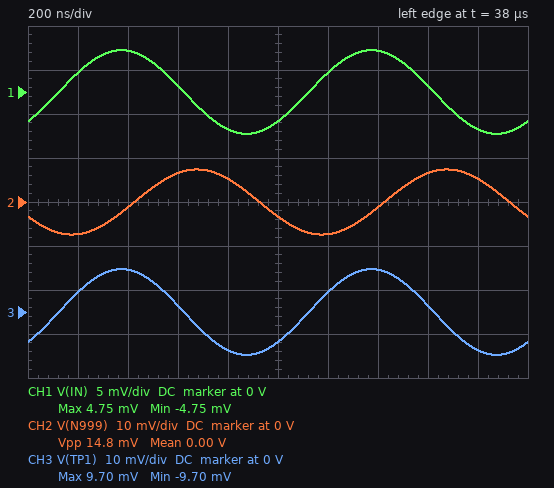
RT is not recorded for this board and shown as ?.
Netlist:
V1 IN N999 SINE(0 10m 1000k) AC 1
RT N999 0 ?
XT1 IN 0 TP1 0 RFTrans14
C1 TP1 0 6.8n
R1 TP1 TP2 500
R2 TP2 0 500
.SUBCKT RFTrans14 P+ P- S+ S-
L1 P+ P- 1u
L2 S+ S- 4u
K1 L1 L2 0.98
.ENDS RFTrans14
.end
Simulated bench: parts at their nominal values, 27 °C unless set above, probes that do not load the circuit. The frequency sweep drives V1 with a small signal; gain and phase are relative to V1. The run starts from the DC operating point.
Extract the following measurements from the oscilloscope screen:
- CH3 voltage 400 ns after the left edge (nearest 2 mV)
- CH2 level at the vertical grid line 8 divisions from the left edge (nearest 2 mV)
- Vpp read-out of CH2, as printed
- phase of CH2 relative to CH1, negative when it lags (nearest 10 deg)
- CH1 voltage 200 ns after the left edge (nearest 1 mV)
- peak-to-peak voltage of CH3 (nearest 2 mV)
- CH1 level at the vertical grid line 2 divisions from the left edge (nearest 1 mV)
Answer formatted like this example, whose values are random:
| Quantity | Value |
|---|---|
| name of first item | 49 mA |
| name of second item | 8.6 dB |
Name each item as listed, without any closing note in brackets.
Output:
| Quantity | Value |
|---|---|
| CH3 voltage 400 ns after the left edge | 10 mV |
| CH2 level at the vertical grid line 8 divisions from the left edge | 6 mV |
| Vpp read-out of CH2, as printed | 14.8 mV |
| phase of CH2 relative to CH1, negative when it lags | -110 deg |
| CH1 voltage 200 ns after the left edge | 2 mV |
| peak-to-peak voltage of CH3 | 20 mV |
| CH1 level at the vertical grid line 2 divisions from the left edge | 5 mV |
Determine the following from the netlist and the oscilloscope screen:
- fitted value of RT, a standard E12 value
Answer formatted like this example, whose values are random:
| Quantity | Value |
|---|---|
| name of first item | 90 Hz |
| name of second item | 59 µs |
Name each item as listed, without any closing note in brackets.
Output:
| Quantity | Value |
|---|---|
| fitted value of RT, a standard E12 value | 120 Ω |
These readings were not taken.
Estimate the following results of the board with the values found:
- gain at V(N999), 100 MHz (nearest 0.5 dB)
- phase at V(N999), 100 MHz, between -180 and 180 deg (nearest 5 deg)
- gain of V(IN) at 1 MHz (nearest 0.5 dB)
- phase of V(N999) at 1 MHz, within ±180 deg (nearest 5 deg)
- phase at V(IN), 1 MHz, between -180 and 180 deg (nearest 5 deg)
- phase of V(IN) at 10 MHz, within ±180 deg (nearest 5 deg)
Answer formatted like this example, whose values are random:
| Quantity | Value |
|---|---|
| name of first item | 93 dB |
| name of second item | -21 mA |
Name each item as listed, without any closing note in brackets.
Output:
| Quantity | Value |
|---|---|
| gain at V(N999), 100 MHz | 0 dB |
| phase at V(N999), 100 MHz, between -180 and 180 deg | 170 deg |
| gain of V(IN) at 1 MHz | -6.5 dB |
| phase of V(N999) at 1 MHz, within ±180 deg | -155 deg |
| phase at V(IN), 1 MHz, between -180 and 180 deg | -45 deg |
| phase of V(IN) at 10 MHz, within ±180 deg | 90 deg |
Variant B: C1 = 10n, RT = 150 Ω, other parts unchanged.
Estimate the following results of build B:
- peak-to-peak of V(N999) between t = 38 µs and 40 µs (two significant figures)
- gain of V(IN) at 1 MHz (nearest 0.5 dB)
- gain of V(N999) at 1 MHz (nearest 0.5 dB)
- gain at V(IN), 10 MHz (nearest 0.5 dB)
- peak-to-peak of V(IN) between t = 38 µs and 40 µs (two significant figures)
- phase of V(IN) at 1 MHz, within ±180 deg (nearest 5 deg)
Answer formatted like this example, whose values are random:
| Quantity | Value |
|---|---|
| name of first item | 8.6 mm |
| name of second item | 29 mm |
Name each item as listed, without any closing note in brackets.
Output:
| Quantity | Value |
|---|---|
| peak-to-peak of V(N999) between t = 38 µs and 40 µs | 20 mV |
| gain of V(IN) at 1 MHz | -23.5 dB |
| gain of V(N999) at 1 MHz | 0 dB |
| gain at V(IN), 10 MHz | -37.0 dB |
| peak-to-peak of V(IN) between t = 38 µs and 40 µs | 1.3 mV |
| phase of V(IN) at 1 MHz, within ±180 deg | -85 deg |
